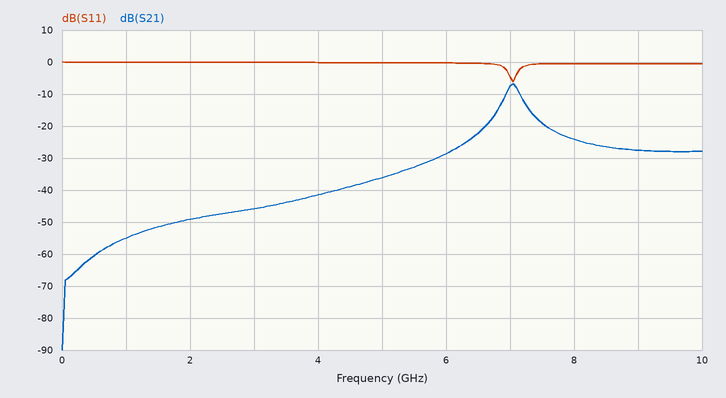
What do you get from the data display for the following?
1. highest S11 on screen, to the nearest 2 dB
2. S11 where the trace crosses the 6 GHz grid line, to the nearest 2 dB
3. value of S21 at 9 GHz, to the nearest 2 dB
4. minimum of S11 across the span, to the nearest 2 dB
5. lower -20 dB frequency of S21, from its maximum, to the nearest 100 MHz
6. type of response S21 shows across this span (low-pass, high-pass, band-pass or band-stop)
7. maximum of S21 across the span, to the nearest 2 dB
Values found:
0 dB
0 dB
-28 dB
-6 dB
6.2 GHz
band-pass
-6 dB
